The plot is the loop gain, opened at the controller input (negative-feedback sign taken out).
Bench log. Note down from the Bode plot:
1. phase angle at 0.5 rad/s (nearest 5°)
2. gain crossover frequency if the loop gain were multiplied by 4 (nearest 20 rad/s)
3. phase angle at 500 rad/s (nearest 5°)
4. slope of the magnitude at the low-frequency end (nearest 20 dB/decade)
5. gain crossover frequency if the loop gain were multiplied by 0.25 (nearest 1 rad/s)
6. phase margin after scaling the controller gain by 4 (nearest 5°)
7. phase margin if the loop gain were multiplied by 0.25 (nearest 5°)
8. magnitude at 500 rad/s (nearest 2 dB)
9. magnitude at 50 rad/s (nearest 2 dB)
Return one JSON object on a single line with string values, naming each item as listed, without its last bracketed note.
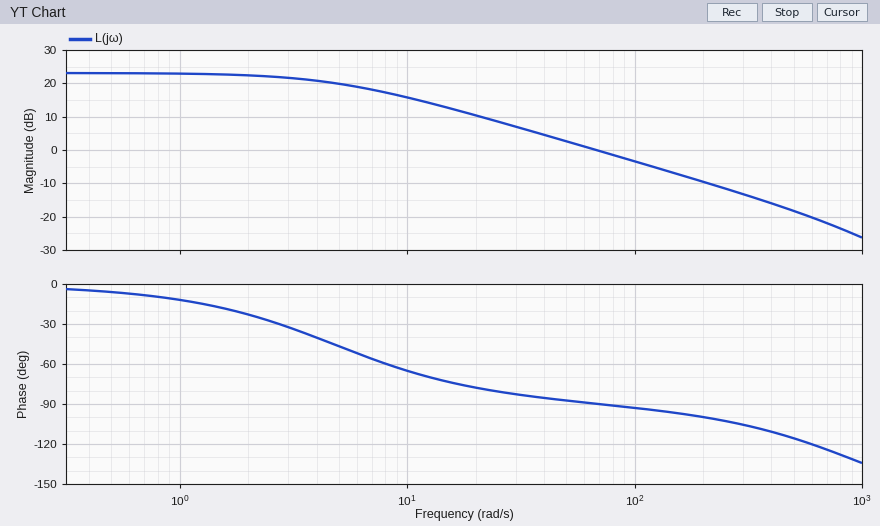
{"phase angle at 0.5 rad/s": "-5°", "gain crossover frequency if the loop gain were multiplied by 4": "260 rad/s", "phase angle at 500 rad/s": "-115°", "slope of the magnitude at the low-frequency end": "0 dB/decade", "gain crossover frequency if the loop gain were multiplied by 0.25": "16 rad/s", "phase margin after scaling the controller gain by 4": "75°", "phase margin if the loop gain were multiplied by 0.25": "105°", "magnitude at 500 rad/s": "-18 dB", "magnitude at 50 rad/s": "2 dB"}
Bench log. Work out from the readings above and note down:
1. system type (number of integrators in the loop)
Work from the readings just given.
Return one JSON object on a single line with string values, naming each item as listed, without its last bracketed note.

{"system type": "0"}
